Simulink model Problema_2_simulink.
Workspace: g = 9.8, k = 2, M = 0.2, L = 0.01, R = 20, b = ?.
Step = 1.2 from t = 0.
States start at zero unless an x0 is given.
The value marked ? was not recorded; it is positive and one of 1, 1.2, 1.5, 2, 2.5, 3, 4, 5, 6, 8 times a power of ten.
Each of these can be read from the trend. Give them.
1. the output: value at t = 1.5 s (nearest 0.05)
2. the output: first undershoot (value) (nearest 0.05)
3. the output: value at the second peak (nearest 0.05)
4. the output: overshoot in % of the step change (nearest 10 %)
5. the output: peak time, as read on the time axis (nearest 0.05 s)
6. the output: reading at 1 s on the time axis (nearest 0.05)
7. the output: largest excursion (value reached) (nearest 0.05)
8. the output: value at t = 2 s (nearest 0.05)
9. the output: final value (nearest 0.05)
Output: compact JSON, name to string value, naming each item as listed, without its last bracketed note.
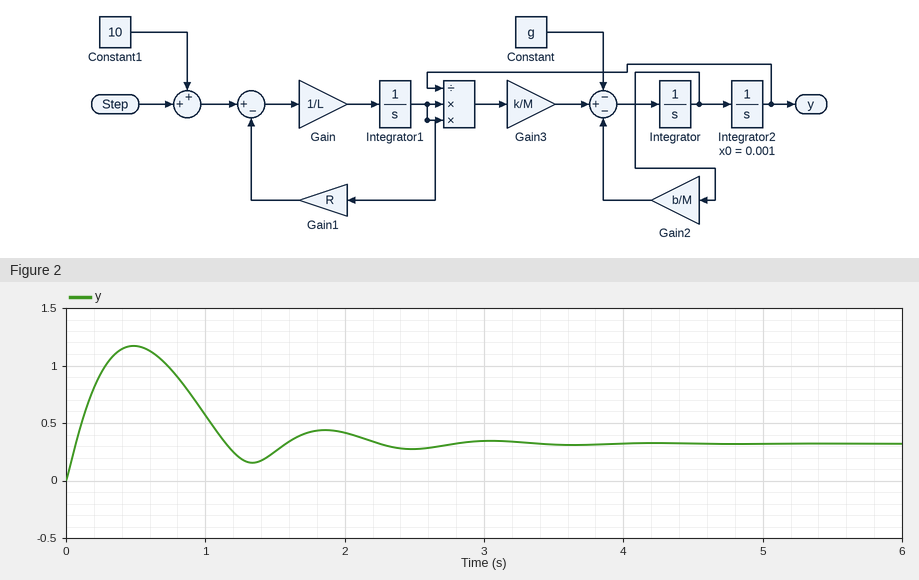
{"the output: value at t = 1.5 s": "0.25", "the output: first undershoot (value)": "0.15", "the output: value at the second peak": "0.45", "the output: overshoot in % of the step change": "270 %", "the output: peak time, as read on the time axis": "0.50 s", "the output: reading at 1 s on the time axis": "0.55", "the output: largest excursion (value reached)": "1.15", "the output: value at t = 2 s": "0.40", "the output: final value": "0.30"}
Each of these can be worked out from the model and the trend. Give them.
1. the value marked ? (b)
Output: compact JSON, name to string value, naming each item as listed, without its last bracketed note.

{"the value marked ?": "0.5"}
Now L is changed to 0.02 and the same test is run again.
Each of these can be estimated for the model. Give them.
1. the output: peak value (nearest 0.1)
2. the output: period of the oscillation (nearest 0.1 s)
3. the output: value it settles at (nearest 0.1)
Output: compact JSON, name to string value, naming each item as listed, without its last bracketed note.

{"the output: peak value": "1.1", "the output: period of the oscillation": "1.4 s", "the output: value it settles at": "0.3"}
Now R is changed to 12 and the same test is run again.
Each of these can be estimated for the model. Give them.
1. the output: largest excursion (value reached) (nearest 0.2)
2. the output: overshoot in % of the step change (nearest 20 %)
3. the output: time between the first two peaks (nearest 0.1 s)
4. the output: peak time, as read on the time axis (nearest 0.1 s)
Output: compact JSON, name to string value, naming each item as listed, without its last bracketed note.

{"the output: largest excursion (value reached)": "2.6", "the output: overshoot in % of the step change": "200 %", "the output: time between the first two peaks": "2.5 s", "the output: peak time, as read on the time axis": "0.7 s"}
